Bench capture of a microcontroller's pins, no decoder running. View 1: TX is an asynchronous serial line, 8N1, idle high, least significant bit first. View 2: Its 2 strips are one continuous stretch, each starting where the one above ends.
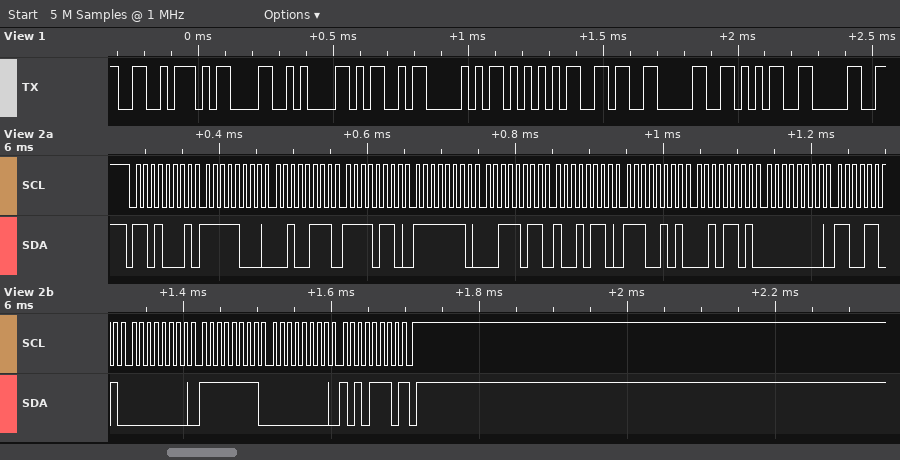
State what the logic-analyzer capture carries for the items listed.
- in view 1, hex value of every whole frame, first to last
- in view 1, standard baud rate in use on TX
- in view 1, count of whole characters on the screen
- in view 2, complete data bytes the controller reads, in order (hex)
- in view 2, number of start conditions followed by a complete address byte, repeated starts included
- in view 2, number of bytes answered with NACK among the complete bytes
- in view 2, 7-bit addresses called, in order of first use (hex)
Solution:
A6 0D 0A 4D 50 55 36 30 35 30
38400 baud
10
F8 27 F6 FE 3B 96 E5 2D 00 CD 00 FF 00 AE
1
1
0x68
